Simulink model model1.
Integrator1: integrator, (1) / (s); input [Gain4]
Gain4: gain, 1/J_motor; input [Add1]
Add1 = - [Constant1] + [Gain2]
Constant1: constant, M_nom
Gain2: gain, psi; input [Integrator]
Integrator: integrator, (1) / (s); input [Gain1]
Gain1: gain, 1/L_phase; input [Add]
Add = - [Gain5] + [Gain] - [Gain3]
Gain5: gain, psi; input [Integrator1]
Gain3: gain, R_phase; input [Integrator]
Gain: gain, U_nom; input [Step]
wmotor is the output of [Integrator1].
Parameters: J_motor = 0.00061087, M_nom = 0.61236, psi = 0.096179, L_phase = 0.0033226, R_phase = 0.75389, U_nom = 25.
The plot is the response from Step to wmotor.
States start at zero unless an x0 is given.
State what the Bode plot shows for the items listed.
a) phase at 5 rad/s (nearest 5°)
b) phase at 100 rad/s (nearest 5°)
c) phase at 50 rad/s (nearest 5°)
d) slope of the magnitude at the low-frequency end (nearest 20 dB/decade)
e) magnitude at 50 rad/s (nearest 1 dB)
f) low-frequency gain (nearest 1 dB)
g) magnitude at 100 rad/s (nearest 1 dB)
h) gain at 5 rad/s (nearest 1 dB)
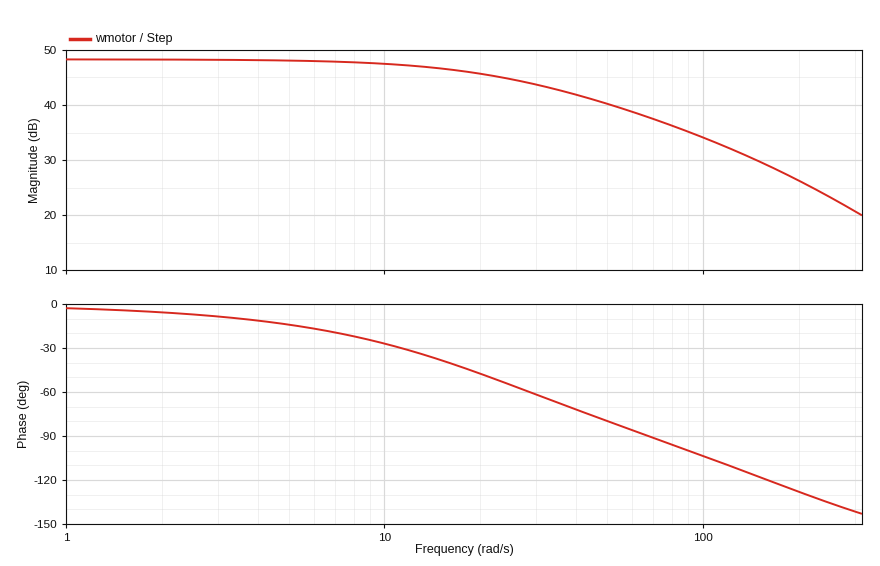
-15°
-105°
-80°
0 dB/decade
40 dB
48 dB
34 dB
48 dB
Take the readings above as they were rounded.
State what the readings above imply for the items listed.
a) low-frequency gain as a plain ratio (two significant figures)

250
